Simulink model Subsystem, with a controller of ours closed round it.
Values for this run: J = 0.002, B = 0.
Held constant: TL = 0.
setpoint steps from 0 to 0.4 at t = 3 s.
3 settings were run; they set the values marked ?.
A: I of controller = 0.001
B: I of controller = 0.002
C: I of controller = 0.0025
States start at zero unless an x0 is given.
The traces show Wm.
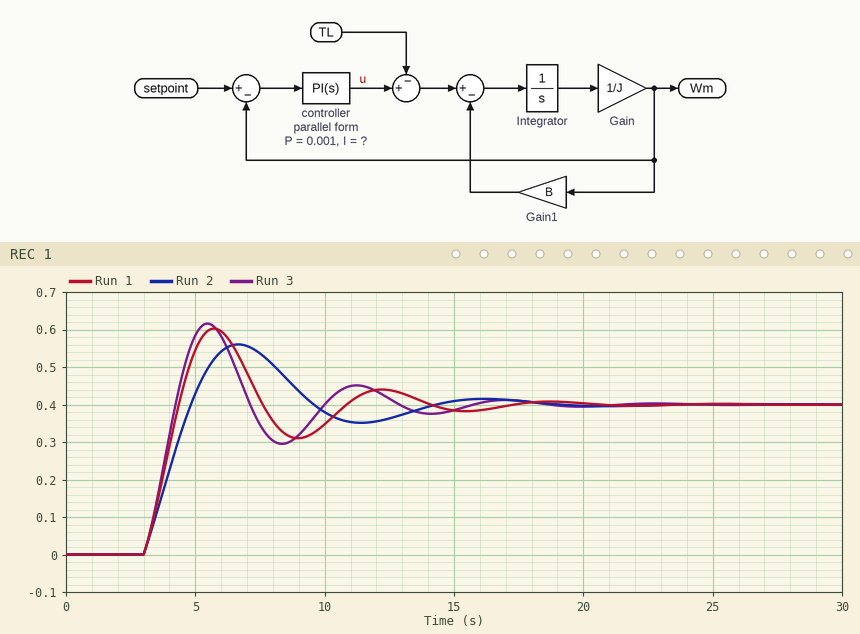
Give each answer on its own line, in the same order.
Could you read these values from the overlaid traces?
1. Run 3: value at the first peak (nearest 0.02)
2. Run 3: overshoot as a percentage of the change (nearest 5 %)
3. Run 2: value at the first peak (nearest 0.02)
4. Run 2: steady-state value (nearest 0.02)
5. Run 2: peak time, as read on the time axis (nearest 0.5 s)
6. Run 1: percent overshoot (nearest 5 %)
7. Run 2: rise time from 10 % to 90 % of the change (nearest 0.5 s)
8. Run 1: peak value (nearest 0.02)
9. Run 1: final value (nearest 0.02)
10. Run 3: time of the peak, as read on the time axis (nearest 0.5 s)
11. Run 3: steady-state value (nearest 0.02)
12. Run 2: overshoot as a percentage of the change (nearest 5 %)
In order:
0.62
55 %
0.56
0.40
6.5 s
50 %
1.5 s
0.60
0.40
5.5 s
0.40
40 %
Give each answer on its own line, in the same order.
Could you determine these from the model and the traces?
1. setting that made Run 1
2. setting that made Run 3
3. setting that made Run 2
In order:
B
C
A
